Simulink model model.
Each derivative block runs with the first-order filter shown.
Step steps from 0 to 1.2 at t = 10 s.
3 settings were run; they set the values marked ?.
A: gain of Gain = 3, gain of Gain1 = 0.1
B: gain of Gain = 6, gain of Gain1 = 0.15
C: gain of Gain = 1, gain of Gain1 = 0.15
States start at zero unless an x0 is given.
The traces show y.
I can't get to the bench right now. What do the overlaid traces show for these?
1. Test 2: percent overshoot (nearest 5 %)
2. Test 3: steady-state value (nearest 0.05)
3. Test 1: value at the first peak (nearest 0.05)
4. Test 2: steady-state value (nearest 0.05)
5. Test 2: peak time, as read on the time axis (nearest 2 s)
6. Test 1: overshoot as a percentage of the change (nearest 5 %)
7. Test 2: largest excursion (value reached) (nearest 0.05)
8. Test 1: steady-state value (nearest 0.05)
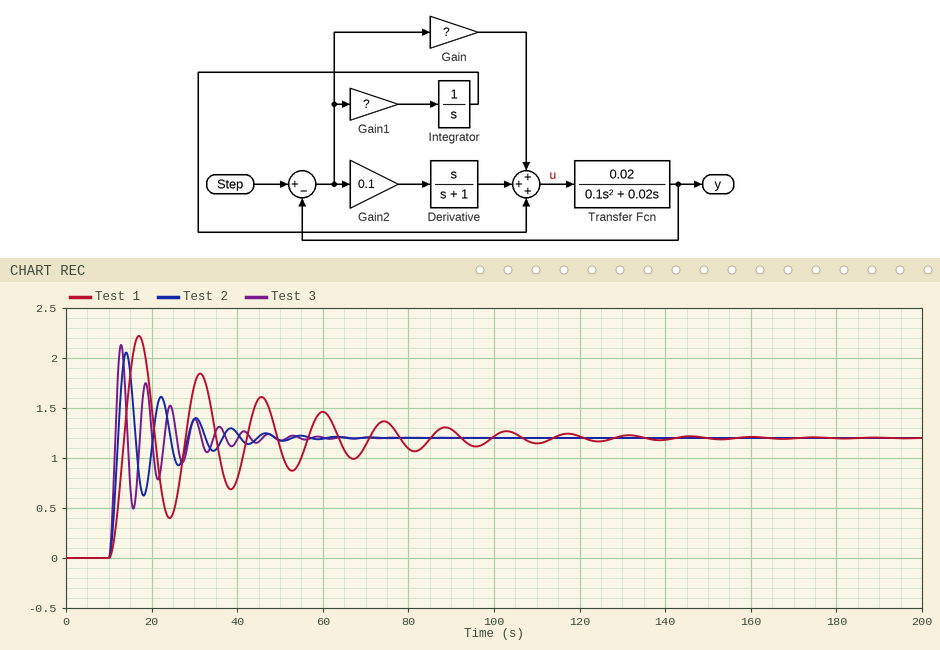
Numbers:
70 %
1.20
2.20
1.20
14 s
85 %
2.05
1.20
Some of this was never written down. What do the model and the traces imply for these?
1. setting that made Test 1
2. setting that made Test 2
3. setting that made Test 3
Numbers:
C
A
B
